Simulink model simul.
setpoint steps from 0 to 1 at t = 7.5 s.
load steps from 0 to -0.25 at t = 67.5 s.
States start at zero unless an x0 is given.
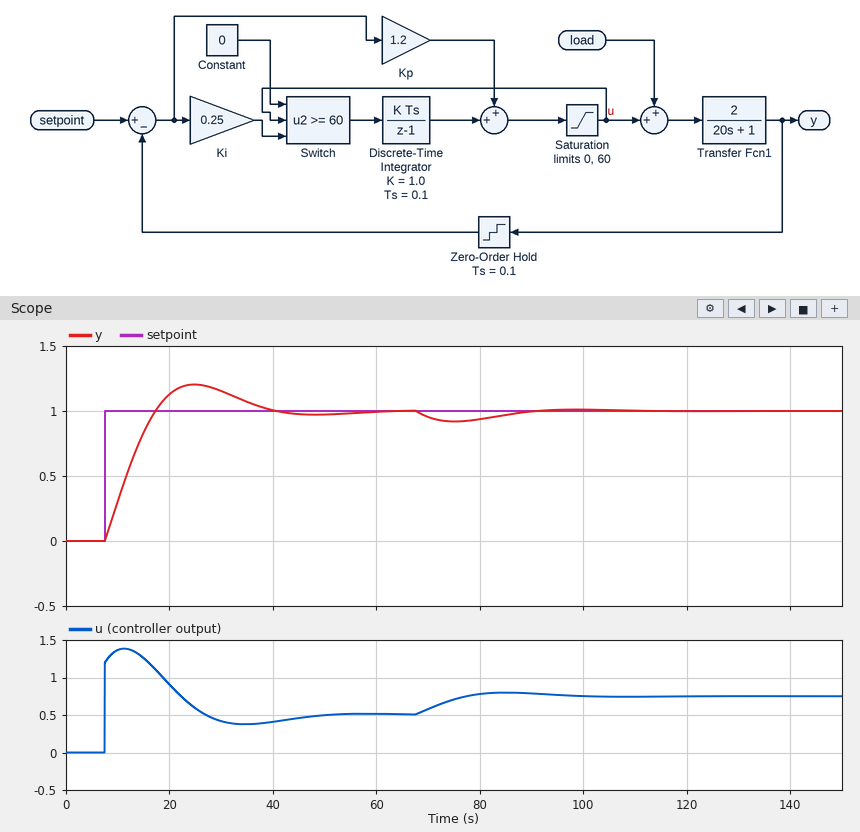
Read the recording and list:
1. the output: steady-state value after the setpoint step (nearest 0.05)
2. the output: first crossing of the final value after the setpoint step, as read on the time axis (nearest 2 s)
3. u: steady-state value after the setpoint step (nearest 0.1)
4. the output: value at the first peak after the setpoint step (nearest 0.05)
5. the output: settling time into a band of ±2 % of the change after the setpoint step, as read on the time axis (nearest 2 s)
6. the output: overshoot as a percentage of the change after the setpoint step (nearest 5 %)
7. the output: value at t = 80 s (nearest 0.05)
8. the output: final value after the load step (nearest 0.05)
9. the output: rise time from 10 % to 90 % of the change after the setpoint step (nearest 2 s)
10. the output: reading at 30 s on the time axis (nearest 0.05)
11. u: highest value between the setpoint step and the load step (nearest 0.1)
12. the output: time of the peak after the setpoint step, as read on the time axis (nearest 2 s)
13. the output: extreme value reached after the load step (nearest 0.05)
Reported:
1.00
18 s
0.5
1.20
54 s
20 %
0.95
1.00
8 s
1.15
1.4
24 s
0.90
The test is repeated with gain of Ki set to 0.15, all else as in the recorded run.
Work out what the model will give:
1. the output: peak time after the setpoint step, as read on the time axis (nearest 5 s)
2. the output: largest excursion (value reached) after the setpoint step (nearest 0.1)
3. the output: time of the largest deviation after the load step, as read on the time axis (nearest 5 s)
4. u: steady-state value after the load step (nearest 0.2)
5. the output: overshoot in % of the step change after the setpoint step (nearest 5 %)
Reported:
30 s
1.1
75 s
0.8
10 %
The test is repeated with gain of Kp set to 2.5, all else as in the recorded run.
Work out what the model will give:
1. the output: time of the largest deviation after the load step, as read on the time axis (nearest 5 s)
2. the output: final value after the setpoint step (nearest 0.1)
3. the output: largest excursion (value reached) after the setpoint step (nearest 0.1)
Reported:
75 s
1.0
1.1
